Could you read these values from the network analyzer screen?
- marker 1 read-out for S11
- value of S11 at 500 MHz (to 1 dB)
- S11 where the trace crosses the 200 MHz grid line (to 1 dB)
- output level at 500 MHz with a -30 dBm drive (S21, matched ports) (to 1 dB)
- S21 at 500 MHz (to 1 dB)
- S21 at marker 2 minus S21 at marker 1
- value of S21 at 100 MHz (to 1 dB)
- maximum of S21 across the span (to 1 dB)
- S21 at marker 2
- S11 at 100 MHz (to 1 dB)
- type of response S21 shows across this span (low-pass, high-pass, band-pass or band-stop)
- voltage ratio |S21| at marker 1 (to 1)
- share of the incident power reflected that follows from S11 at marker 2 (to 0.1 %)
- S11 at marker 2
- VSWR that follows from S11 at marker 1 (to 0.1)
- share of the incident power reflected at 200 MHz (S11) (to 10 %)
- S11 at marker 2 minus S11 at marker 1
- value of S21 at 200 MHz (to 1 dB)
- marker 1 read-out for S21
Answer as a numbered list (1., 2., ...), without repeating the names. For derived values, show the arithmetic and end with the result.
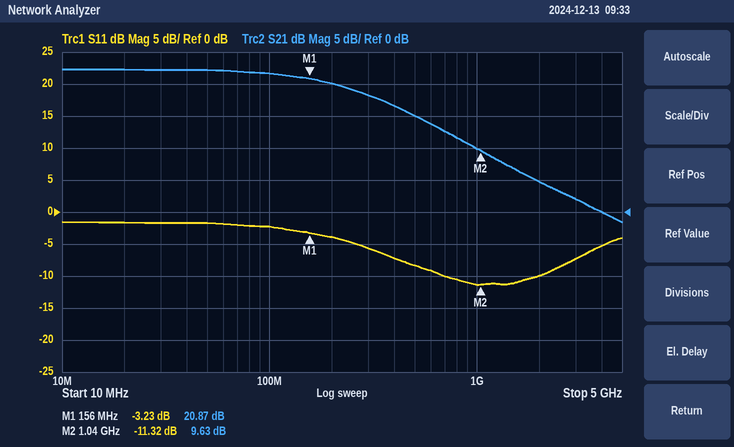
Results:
1. -3.23 dB
2. -8 dB
3. -4 dB
4. -30 dBm + (15 dB) = -15 dBm
5. 15 dB
6. 9.63 − (20.87) = -11.24 dB
7. 22 dB
8. 22 dB
9. 9.63 dB
10. -2 dB
11. low-pass
12. 10^(20.87/20) ≈ 11
13. 10^(-11.32/10) ≈ 7.4 %
14. -11.32 dB
15. (1 + 0.6894)/(1 − 0.6894) ≈ 5.4
16. 10^(-4/10) ≈ 40 %
17. -11.32 − (-3.23) = -8.09 dB
18. 20 dB
19. 20.87 dB
